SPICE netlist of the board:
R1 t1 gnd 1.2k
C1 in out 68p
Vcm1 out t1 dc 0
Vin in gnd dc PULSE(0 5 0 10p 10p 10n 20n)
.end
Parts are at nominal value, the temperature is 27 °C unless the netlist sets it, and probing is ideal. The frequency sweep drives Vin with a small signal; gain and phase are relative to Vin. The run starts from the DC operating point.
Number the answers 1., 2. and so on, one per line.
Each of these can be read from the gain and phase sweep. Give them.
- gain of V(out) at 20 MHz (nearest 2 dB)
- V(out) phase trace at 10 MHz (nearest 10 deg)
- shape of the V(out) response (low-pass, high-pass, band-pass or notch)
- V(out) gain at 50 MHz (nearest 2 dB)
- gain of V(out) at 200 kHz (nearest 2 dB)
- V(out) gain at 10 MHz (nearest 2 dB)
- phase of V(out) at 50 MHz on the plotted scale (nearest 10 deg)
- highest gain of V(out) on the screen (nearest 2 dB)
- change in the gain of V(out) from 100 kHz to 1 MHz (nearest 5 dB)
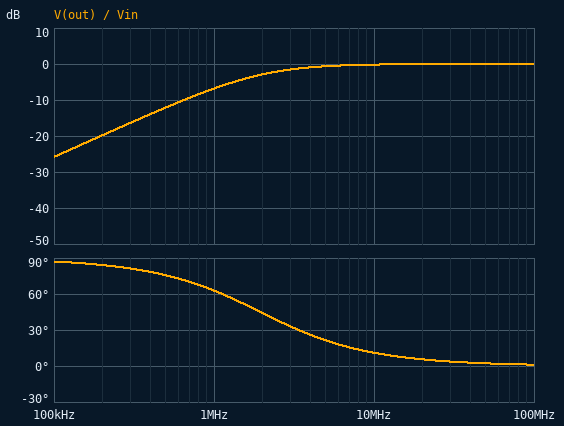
1. 0 dB
2. 10 deg
3. high-pass
4. 0 dB
5. -20 dB
6. 0 dB
7. 0 deg
8. 0 dB
9. 20 dB
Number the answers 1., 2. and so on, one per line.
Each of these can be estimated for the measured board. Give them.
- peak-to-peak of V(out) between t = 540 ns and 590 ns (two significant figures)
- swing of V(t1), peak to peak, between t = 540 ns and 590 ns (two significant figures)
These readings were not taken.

1. 5.3 V
2. 5.3 V
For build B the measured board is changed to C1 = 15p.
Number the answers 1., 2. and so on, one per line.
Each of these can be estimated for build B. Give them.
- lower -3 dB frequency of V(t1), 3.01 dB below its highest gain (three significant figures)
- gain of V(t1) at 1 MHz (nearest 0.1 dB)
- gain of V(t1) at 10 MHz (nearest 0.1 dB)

1. 8.84 MHz
2. -19.0 dB
3. -2.5 dB
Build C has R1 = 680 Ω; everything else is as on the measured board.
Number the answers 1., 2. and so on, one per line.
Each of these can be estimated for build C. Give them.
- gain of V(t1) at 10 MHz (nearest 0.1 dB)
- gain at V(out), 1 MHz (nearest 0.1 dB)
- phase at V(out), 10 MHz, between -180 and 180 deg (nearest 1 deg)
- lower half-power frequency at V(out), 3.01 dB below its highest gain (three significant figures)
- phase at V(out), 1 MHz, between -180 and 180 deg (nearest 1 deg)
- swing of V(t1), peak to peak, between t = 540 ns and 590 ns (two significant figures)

1. -0.5 dB
2. -11.1 dB
3. 19 deg
4. 3.44 MHz
5. 74 deg
6. 5.5 V
